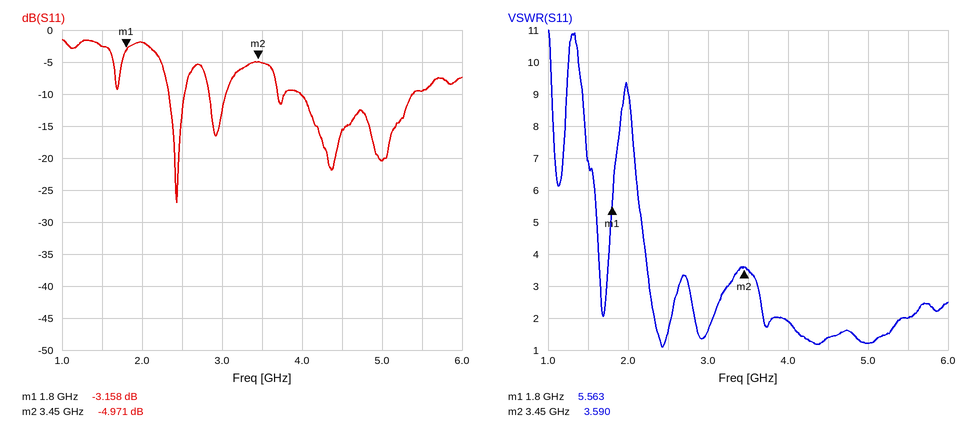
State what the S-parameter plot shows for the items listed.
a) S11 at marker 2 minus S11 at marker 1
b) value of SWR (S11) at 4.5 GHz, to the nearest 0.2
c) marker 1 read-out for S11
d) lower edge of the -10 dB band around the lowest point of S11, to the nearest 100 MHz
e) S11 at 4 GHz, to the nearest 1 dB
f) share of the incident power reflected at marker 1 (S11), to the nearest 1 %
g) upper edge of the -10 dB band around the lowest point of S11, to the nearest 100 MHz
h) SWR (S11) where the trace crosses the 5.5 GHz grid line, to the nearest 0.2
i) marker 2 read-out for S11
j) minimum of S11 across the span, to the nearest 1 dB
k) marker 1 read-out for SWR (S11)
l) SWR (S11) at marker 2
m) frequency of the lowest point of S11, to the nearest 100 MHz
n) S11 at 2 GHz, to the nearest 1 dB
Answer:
-1.813 dB
1.4
-3.158 dB
2.3 GHz
-10 dB
48 %
2.5 GHz
2.0
-4.971 dB
-27 dB
5.563
3.590
2.4 GHz
-2 dB
